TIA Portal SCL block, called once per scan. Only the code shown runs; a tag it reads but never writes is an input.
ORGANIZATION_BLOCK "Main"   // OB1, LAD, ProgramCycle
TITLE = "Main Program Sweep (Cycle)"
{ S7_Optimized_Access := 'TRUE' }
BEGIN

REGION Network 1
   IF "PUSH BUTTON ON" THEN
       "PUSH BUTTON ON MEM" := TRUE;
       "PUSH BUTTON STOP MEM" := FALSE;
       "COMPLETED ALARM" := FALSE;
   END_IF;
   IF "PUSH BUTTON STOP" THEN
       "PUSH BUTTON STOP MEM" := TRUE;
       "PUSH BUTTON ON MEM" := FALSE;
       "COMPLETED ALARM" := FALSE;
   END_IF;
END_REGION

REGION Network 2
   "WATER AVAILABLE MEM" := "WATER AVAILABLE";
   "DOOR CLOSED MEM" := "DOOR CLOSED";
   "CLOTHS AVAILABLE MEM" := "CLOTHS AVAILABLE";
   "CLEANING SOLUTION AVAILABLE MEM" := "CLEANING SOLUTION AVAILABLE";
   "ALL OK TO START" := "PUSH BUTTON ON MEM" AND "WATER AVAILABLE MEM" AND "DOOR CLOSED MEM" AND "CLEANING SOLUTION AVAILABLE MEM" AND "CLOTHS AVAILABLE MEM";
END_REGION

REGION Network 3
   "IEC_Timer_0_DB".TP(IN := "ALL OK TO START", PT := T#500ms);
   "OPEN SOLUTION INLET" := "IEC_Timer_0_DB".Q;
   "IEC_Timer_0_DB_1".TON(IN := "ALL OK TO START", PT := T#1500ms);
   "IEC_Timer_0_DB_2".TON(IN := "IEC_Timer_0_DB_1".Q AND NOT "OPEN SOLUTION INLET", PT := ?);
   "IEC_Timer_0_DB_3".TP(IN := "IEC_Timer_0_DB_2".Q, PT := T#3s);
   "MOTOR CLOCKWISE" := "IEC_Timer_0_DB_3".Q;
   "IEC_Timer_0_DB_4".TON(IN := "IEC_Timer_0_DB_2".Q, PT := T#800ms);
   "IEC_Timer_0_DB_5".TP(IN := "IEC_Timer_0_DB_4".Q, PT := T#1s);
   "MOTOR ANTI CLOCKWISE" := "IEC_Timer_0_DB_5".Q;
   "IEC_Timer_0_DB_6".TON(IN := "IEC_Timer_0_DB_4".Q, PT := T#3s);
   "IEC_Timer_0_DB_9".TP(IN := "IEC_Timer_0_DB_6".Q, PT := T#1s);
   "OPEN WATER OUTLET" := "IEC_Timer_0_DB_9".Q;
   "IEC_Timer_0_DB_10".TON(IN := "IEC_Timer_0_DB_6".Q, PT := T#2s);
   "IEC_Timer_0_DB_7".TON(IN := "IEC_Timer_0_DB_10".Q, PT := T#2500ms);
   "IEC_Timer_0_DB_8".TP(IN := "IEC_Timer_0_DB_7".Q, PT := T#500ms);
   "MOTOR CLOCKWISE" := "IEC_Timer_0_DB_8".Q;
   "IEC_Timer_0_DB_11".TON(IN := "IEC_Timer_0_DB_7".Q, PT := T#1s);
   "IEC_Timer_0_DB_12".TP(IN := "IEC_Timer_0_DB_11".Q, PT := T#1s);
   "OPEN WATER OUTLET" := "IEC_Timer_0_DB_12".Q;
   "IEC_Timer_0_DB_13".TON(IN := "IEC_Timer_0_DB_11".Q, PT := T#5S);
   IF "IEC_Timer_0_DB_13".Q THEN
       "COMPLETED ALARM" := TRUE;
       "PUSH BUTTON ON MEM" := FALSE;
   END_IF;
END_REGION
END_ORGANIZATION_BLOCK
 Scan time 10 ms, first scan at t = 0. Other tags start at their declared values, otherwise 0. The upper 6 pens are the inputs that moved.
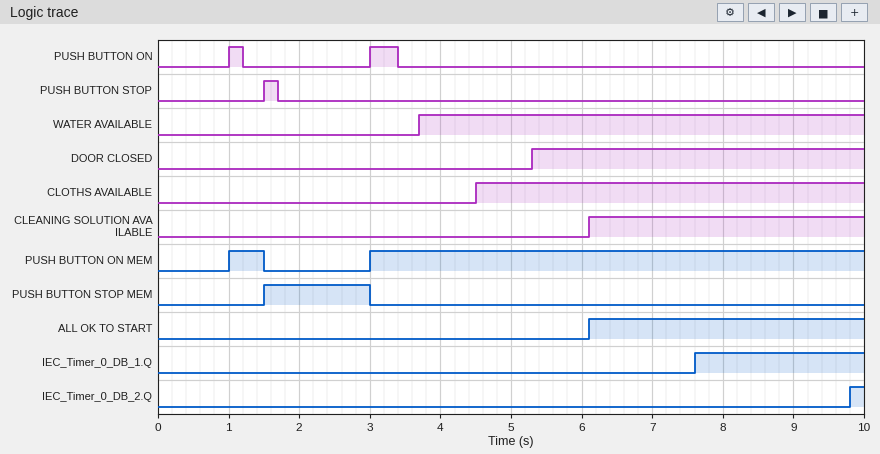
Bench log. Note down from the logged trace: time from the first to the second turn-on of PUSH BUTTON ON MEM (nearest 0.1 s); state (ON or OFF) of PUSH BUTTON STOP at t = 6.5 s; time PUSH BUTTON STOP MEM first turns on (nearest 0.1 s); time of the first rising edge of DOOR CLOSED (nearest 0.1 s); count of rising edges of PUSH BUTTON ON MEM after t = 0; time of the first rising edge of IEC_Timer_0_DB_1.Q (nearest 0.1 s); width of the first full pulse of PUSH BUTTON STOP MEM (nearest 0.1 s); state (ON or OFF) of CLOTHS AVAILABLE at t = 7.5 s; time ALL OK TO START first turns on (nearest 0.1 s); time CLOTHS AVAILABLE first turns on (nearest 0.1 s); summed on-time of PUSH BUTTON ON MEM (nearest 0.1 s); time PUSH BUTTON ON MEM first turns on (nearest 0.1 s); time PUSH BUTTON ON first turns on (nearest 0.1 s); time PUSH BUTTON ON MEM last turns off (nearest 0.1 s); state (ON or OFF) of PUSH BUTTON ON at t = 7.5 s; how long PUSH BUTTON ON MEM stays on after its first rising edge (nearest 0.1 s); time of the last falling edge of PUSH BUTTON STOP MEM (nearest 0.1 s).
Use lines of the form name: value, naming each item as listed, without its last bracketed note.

time from the first to the second turn-on of PUSH BUTTON ON MEM: 2.0 s
state (ON or OFF) of PUSH BUTTON STOP at t = 6.5 s: OFF
time PUSH BUTTON STOP MEM first turns on: 1.5 s
time of the first rising edge of DOOR CLOSED: 5.3 s
count of rising edges of PUSH BUTTON ON MEM after t = 0: 2
time of the first rising edge of IEC_Timer_0_DB_1.Q: 7.6 s
width of the first full pulse of PUSH BUTTON STOP MEM: 1.5 s
state (ON or OFF) of CLOTHS AVAILABLE at t = 7.5 s: ON
time ALL OK TO START first turns on: 6.1 s
time CLOTHS AVAILABLE first turns on: 4.5 s
summed on-time of PUSH BUTTON ON MEM: 7.5 s
time PUSH BUTTON ON MEM first turns on: 1.0 s
time PUSH BUTTON ON first turns on: 1.0 s
time PUSH BUTTON ON MEM last turns off: 1.5 s
state (ON or OFF) of PUSH BUTTON ON at t = 7.5 s: OFF
how long PUSH BUTTON ON MEM stays on after its first rising edge: 0.5 s
time of the last falling edge of PUSH BUTTON STOP MEM: 3.0 s
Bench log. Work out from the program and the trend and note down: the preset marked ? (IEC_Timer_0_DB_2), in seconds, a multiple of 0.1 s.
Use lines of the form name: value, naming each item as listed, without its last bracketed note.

the preset marked ? (IEC_Timer_0_DB_2), in seconds, a multiple of 0.1 s: 2.2 s
